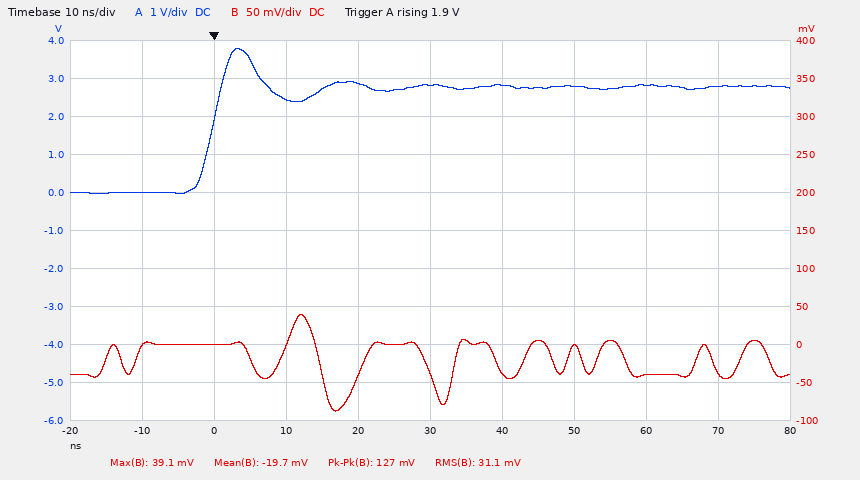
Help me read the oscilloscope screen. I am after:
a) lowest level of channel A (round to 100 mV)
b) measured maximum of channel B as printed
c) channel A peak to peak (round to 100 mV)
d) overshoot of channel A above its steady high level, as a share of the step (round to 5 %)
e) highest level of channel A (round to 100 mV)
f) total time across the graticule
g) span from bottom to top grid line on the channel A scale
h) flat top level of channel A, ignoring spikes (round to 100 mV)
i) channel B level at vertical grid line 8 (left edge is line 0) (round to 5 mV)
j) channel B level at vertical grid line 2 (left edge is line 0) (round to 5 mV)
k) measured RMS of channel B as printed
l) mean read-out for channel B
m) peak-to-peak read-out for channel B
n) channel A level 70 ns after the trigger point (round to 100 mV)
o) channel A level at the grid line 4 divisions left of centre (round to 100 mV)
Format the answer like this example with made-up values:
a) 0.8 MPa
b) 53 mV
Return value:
a) 0.0 V
b) 39.1 mV
c) 3.8 V
d) 35 %
e) 3.8 V
f) 100 ns
g) 10 V
h) 2.8 V
i) -40 mV
j) 0 mV
k) 31.1 mV
l) -19.7 mV
m) 127 mV
n) 2.8 V
o) 0.0 V
